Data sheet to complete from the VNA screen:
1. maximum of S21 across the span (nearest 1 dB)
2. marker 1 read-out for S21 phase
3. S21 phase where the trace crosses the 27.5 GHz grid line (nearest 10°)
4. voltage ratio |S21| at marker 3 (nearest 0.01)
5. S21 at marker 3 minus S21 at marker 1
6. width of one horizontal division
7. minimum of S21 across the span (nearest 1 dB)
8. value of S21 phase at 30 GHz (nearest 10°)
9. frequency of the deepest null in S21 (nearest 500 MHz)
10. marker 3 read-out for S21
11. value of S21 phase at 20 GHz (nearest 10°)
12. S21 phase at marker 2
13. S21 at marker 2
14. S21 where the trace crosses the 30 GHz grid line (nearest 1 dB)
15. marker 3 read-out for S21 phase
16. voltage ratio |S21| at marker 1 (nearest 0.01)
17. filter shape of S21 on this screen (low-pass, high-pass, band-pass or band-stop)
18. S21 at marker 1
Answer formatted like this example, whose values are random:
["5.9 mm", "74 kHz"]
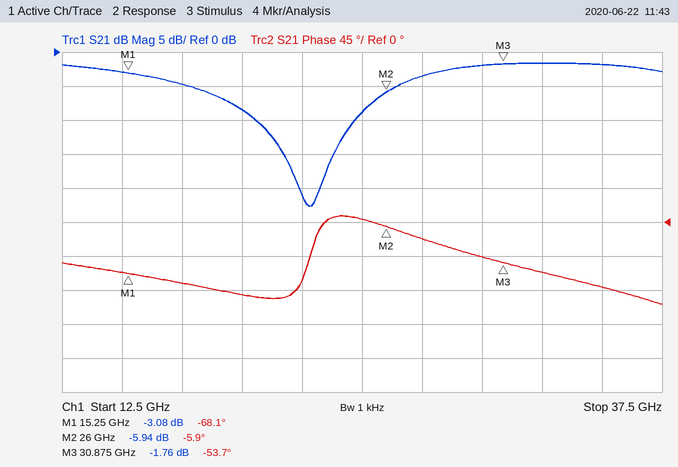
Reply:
["-2 dB", "-68.1°", "-20°", "0.82", "1.32 dB", "2.5 GHz", "-23 dB", "-50°", "23.0 GHz", "-1.76 dB", "-100°", "-5.9°", "-5.94 dB", "-2 dB", "-53.7°", "0.70", "band-stop", "-3.08 dB"]
